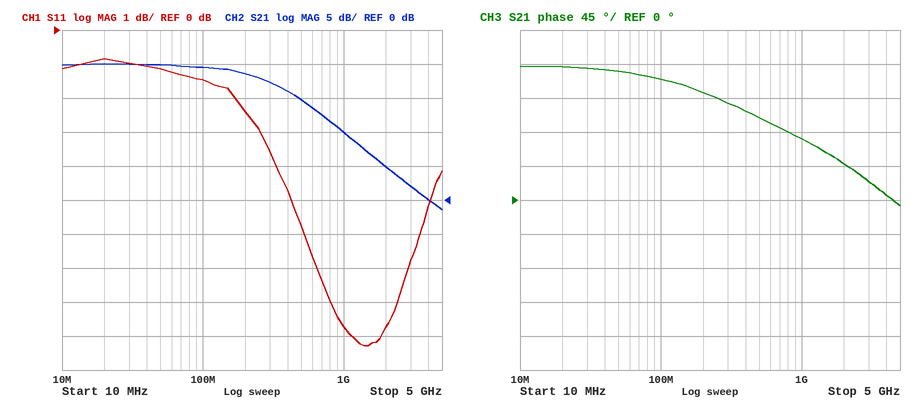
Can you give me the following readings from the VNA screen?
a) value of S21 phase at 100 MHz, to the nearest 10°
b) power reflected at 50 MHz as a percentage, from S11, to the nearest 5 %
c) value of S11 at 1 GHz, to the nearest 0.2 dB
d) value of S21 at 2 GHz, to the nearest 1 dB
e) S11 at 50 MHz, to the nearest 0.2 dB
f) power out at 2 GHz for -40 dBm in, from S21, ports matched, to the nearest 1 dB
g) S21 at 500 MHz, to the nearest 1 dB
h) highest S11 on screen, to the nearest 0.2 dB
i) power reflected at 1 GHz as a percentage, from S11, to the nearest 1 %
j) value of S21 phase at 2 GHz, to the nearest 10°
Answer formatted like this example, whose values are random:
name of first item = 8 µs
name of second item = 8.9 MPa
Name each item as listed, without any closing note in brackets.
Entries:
value of S21 phase at 100 MHz, to the nearest 10° = 160°
power reflected at 50 MHz as a percentage, from S11, to the nearest 5 % = 75 %
value of S11 at 1 GHz, to the nearest 0.2 dB = -8.8 dB
value of S21 at 2 GHz, to the nearest 1 dB = 5 dB
S11 at 50 MHz, to the nearest 0.2 dB = -1.2 dB
power out at 2 GHz for -40 dBm in, from S21, ports matched, to the nearest 1 dB = -35 dBm
S21 at 500 MHz, to the nearest 1 dB = 15 dB
highest S11 on screen, to the nearest 0.2 dB = -0.8 dB
power reflected at 1 GHz as a percentage, from S11, to the nearest 1 % = 13 %
value of S21 phase at 2 GHz, to the nearest 10° = 50°
